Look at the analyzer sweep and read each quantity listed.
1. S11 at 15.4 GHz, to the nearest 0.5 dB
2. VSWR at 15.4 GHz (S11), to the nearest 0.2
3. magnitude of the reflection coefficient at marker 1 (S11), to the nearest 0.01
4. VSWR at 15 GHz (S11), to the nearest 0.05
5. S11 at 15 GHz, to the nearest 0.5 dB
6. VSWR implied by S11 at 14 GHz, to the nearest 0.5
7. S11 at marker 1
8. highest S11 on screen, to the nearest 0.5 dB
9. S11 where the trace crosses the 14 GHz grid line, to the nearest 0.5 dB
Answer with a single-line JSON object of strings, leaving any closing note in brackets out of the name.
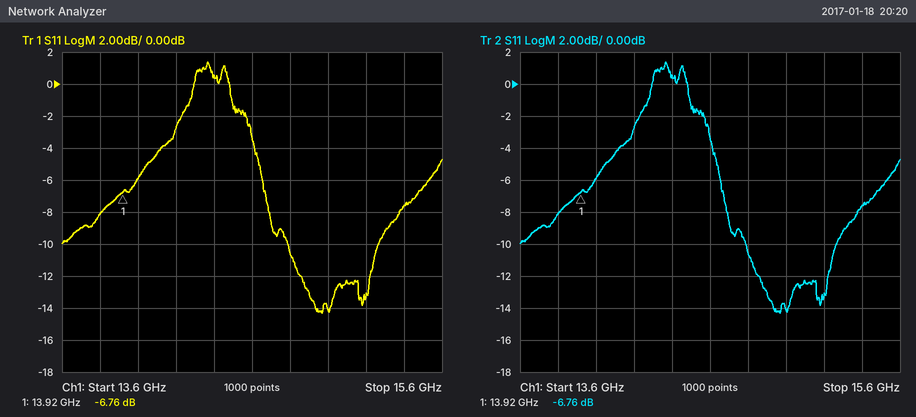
{"S11 at 15.4 GHz, to the nearest 0.5 dB": "-7.5 dB", "VSWR at 15.4 GHz (S11), to the nearest 0.2": "2.4", "magnitude of the reflection coefficient at marker 1 (S11), to the nearest 0.01": "0.46", "VSWR at 15 GHz (S11), to the nearest 0.05": "1.50", "S11 at 15 GHz, to the nearest 0.5 dB": "-14.0 dB", "VSWR implied by S11 at 14 GHz, to the nearest 0.5": "3.0", "S11 at marker 1": "-6.76 dB", "highest S11 on screen, to the nearest 0.5 dB": "1.5 dB", "S11 where the trace crosses the 14 GHz grid line, to the nearest 0.5 dB": "-6.0 dB"}
